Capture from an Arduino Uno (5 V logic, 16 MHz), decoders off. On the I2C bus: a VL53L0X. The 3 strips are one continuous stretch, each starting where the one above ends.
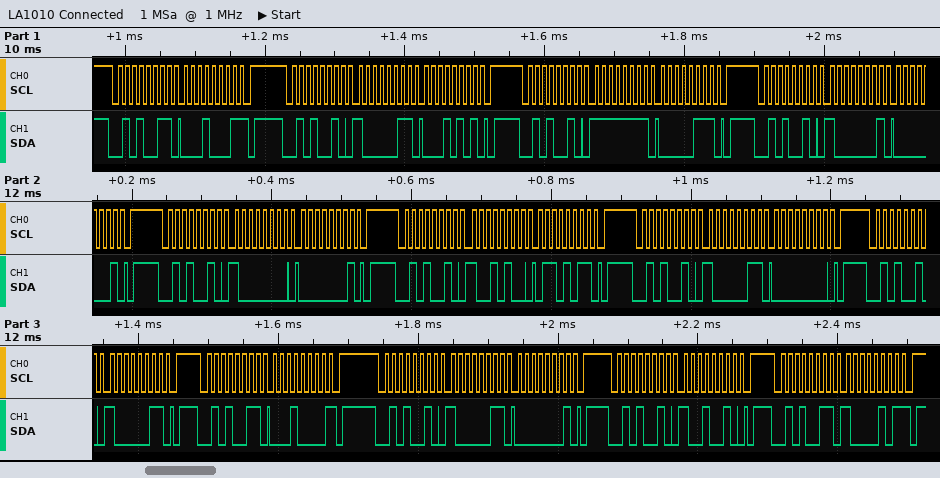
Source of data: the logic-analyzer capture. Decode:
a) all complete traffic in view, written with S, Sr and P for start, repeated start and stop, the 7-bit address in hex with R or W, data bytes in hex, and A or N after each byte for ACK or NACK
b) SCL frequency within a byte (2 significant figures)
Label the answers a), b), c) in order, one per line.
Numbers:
a) S 29R A 11 N P S 29W A 83 A 15 A P S 29W A FF A 07 A P S 29W A 81 A 01 A P S 29W A 80 A 01 A P S 29W A 94 A 6B A P S 29W A 83 A 00 A P S 29W A 83 A P S 29R A 10 N P S 29W A 83 A 01 A P S 29W A 92 A P S 29R A 85 N P
b) 100 kHz
